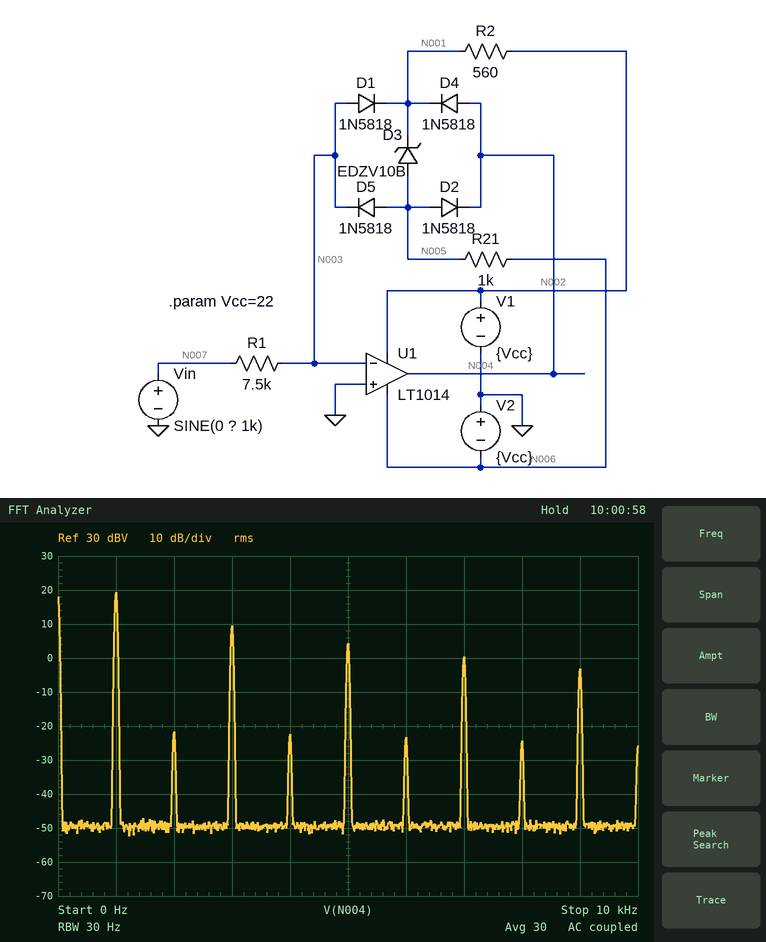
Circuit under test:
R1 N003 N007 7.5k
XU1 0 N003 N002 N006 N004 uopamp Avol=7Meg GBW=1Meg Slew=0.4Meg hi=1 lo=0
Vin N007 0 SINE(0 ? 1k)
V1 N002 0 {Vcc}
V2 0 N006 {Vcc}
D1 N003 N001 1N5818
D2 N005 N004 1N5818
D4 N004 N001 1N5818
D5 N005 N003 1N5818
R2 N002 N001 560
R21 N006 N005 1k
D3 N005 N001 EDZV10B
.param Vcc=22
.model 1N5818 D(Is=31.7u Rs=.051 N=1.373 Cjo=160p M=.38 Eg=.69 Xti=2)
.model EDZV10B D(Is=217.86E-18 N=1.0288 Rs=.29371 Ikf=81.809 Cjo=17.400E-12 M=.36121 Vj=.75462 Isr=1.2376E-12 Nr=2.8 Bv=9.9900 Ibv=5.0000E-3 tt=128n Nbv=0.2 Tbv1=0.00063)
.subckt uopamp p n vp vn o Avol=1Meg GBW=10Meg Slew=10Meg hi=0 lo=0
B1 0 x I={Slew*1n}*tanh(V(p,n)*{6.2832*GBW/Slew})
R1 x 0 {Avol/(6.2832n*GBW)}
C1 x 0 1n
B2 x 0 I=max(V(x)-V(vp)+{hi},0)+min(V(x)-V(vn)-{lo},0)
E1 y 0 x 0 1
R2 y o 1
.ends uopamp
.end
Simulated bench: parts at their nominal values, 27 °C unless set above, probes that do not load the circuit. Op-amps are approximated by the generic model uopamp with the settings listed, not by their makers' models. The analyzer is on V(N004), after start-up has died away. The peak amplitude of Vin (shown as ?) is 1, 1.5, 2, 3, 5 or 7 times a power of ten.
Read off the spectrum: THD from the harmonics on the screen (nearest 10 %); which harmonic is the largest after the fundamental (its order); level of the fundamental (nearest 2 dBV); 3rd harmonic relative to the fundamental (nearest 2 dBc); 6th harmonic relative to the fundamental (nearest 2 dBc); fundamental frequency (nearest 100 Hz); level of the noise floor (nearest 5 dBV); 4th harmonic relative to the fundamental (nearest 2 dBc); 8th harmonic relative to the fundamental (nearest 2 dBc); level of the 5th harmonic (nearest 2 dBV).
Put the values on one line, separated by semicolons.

40 %; 3; 20 dBV; -10 dBc; -42 dBc; 1.0 kHz; -50 dBV; -42 dBc; -44 dBc; 4 dBV
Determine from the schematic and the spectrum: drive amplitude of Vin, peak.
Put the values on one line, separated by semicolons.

10 V
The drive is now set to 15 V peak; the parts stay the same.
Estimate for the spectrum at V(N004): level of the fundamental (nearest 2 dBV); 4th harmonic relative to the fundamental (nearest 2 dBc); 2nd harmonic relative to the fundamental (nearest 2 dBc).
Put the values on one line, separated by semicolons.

20 dBV; -46 dBc; -44 dBc
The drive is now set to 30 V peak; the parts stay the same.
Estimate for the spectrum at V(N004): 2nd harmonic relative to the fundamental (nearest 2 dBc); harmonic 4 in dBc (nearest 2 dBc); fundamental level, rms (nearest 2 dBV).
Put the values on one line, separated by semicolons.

-50 dBc; -52 dBc; 20 dBV
